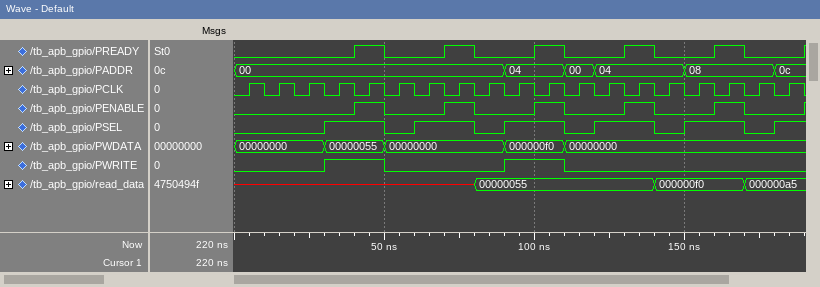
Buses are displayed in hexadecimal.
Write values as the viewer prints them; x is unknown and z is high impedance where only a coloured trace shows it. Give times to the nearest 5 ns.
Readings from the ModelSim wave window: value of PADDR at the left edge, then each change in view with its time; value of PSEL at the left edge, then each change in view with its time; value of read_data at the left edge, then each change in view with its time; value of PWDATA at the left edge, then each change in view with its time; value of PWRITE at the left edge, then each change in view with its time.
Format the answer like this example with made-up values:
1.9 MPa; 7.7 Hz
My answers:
00, 04 at 90 ns, 00 at 110 ns, 04 at 120 ns, 08 at 150 ns, 0c at 180 ns; 0, 1 at 30 ns, 0 at 50 ns, 1 at 60 ns, 0 at 80 ns, 1 at 90 ns, 0 at 110 ns, 1 at 120 ns, 0 at 140 ns, 1 at 150 ns, 0 at 170 ns, 1 at 180 ns; x, 00000055 at 80 ns, 000000f0 at 140 ns, 000000a5 at 170 ns; 00000000, 00000055 at 30 ns, 00000000 at 50 ns, 000000f0 at 90 ns, 00000000 at 110 ns; 0, 1 at 30 ns, 0 at 50 ns, 1 at 90 ns, 0 at 110 ns
